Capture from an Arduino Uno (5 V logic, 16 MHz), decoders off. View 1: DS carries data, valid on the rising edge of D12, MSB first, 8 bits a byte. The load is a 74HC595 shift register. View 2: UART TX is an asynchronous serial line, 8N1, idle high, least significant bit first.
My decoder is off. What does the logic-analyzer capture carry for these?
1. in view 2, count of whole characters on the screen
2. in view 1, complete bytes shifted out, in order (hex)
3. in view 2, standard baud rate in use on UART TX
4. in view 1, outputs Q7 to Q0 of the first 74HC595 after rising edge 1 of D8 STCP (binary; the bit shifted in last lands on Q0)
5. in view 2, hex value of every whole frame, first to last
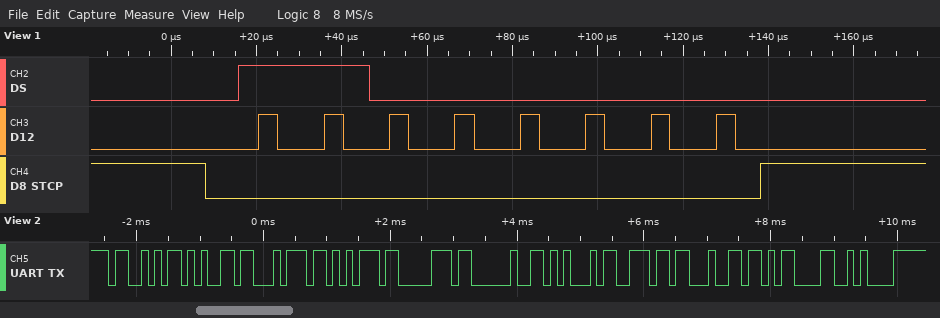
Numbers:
11
0xC0
9600 baud
11000000
0x53 0x65 0x74 0x75 0x70 0x20 0x45 0x6E 0x64 0x0D 0x0A
